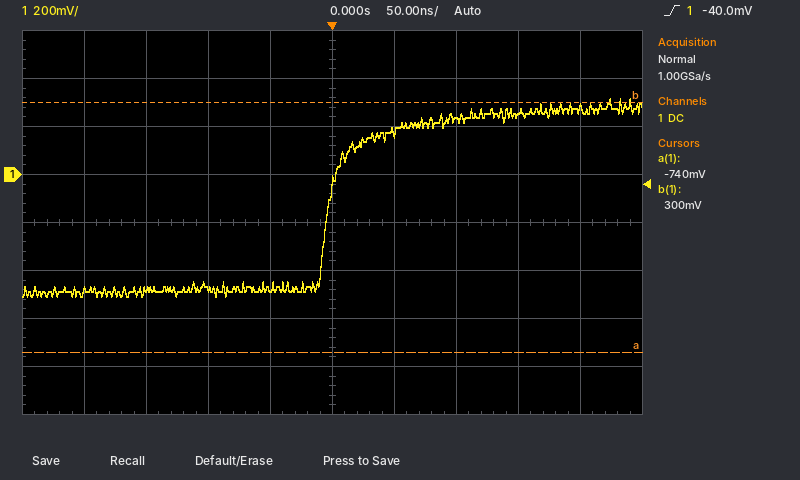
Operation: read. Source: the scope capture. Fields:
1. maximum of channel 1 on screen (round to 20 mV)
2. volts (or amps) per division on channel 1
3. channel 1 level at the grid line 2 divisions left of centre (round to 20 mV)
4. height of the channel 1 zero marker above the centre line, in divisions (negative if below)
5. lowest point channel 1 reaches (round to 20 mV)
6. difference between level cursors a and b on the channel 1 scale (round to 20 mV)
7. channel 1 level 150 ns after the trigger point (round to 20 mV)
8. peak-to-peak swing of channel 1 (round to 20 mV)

320 mV
200 mV
-480 mV
+1.0 div
-500 mV
1.04 V
260 mV
820 mV
